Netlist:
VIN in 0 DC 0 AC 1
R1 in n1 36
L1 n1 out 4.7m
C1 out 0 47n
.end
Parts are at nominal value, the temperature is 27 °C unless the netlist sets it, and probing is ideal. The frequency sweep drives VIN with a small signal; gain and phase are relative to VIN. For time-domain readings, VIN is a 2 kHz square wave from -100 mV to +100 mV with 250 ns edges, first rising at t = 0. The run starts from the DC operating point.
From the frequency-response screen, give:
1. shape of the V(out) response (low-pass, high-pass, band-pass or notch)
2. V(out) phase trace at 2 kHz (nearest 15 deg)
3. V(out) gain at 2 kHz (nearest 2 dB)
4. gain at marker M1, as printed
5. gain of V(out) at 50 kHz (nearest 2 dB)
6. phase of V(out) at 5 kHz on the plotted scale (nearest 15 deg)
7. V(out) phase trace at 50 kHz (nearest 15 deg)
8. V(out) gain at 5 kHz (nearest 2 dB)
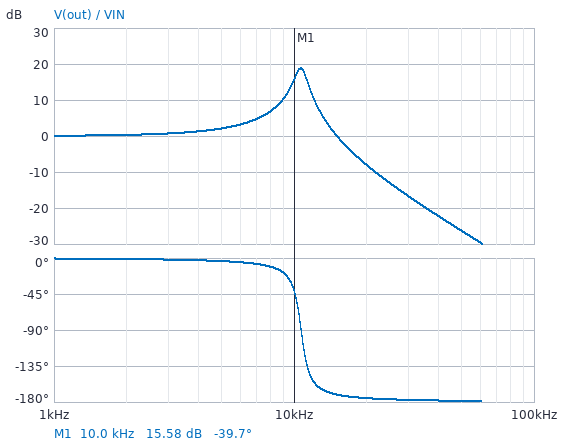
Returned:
low-pass
0 deg
0 dB
15.58 dB
-26 dB
0 deg
-180 deg
2 dB
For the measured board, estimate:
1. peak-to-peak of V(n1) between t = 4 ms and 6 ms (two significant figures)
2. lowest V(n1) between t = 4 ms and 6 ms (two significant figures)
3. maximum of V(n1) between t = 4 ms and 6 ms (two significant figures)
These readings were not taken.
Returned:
240 mV
-120 mV
120 mV
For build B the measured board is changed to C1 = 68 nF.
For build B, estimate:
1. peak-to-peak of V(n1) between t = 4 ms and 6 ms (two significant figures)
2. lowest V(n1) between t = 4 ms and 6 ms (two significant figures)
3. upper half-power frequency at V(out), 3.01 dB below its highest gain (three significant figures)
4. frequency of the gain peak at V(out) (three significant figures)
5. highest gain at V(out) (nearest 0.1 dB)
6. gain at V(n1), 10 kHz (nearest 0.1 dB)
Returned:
230 mV
-120 mV
9.45 kHz
8.86 kHz
17.3 dB
-1.3 dB
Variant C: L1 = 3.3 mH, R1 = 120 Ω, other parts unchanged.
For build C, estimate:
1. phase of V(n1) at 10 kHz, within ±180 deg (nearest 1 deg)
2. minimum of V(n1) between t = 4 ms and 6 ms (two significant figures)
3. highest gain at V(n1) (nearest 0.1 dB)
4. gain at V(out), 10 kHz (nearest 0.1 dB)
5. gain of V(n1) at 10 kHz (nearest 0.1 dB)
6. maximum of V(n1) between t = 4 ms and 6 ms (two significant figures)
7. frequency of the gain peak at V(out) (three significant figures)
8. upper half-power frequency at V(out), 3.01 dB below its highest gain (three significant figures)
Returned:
-42 deg
-130 mV
0 dB
5.6 dB
-2.6 dB
130 mV
12.1 kHz
14.8 kHz
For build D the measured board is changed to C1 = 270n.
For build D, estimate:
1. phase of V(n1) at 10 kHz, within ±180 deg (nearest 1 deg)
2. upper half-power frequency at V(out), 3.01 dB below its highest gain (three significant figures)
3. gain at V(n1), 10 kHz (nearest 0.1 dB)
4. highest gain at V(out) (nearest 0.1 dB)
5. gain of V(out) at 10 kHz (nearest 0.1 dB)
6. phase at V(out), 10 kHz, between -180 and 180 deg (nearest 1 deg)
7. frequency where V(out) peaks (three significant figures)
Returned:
9 deg
4.96 kHz
-0.1 dB
11.4 dB
-12.2 dB
-171 deg
4.38 kHz
